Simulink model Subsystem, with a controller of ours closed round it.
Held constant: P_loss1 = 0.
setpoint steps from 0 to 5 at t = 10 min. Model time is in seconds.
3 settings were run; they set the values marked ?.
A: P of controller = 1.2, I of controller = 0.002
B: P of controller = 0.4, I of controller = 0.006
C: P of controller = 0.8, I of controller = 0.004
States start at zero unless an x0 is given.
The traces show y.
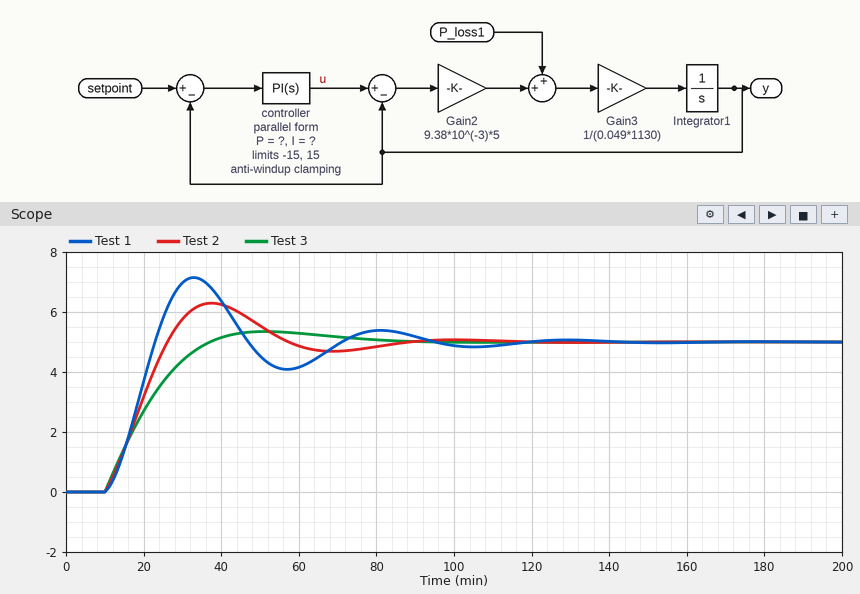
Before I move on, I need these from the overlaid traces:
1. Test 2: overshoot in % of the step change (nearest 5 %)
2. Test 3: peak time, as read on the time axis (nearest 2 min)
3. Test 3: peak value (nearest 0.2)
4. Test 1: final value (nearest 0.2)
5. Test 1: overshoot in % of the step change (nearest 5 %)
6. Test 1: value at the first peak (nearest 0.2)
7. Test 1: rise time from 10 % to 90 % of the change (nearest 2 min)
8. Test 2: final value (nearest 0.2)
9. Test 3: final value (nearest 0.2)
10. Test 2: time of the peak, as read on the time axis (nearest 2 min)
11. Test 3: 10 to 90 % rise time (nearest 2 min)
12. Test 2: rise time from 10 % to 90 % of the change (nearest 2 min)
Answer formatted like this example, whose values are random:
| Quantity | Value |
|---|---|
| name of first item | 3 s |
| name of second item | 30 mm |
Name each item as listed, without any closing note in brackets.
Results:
| Quantity | Value |
|---|---|
| Test 2: overshoot in % of the step change | 25 % |
| Test 3: peak time, as read on the time axis | 52 min |
| Test 3: peak value | 5.4 |
| Test 1: final value | 5.0 |
| Test 1: overshoot in % of the step change | 45 % |
| Test 1: value at the first peak | 7.2 |
| Test 1: rise time from 10 % to 90 % of the change | 10 min |
| Test 2: final value | 5.0 |
| Test 3: final value | 5.0 |
| Test 2: time of the peak, as read on the time axis | 38 min |
| Test 3: 10 to 90 % rise time | 20 min |
| Test 2: rise time from 10 % to 90 % of the change | 12 min |
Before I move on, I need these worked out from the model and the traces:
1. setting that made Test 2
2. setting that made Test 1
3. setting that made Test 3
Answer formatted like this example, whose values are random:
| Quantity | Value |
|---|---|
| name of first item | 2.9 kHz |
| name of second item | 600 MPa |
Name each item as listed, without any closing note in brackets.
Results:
| Quantity | Value |
|---|---|
| setting that made Test 2 | C |
| setting that made Test 1 | B |
| setting that made Test 3 | A |
